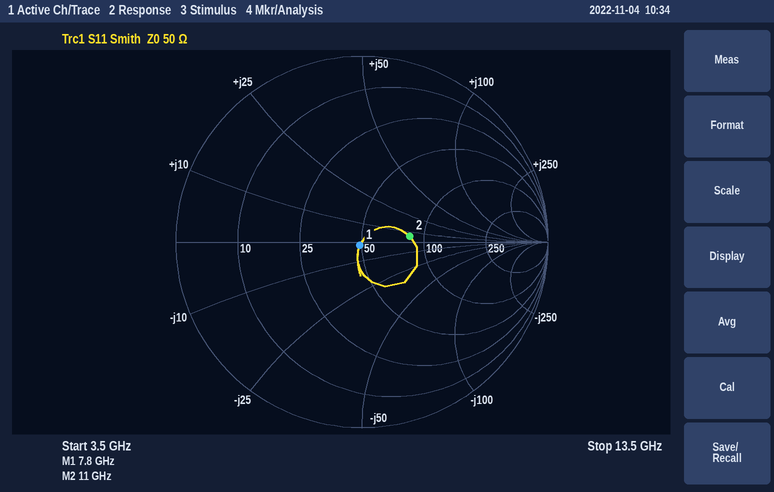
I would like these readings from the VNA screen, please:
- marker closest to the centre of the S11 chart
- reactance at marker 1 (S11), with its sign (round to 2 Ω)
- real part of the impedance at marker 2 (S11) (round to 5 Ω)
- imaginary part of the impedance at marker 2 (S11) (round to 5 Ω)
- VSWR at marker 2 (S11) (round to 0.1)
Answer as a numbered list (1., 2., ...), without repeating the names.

1. marker 1
2. -2 Ω
3. 85 Ω
4. +5 Ω
5. 1.7
